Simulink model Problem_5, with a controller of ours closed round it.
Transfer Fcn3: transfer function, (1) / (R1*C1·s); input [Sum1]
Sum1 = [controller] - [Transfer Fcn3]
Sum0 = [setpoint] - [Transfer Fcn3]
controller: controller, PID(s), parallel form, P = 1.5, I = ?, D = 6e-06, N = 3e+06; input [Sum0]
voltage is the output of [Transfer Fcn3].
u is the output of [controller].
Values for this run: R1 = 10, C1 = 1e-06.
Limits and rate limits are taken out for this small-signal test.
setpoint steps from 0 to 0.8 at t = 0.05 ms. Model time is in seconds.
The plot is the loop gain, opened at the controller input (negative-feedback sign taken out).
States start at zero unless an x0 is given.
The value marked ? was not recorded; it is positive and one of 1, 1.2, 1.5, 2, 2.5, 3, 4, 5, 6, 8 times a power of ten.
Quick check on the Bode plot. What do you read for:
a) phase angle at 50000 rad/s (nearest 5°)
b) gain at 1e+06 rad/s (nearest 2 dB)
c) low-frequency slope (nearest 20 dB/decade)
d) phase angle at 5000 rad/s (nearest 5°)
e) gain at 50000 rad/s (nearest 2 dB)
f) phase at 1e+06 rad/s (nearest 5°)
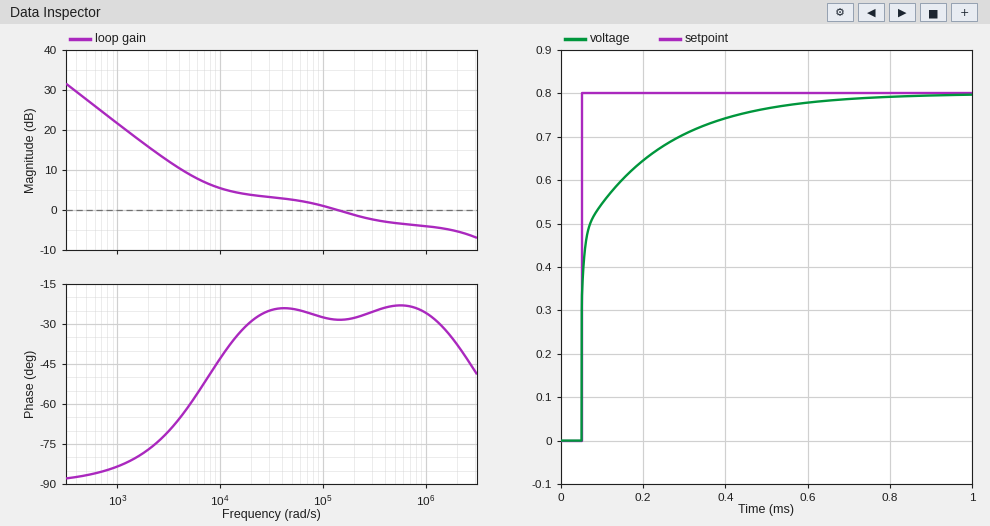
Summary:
-25°
-4 dB
-20 dB/decade
-60°
2 dB
-25°
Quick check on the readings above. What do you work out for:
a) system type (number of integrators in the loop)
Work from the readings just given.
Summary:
1
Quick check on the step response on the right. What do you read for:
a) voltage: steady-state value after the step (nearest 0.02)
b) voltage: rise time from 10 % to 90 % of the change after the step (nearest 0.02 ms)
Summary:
0.80
0.28 ms
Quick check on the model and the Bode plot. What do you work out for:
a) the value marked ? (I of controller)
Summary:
12000
